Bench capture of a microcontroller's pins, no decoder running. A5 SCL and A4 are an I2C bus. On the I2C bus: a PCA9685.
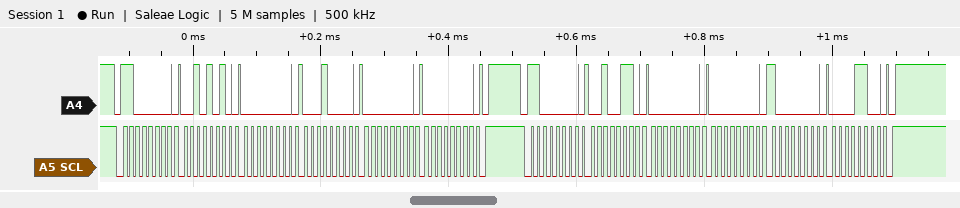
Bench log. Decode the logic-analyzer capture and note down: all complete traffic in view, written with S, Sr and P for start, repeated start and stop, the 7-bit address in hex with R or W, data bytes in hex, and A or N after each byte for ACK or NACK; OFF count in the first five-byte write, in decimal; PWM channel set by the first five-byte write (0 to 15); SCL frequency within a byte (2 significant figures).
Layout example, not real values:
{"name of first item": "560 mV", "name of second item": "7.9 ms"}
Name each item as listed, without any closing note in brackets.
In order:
{"all complete traffic in view, written with S, Sr and P for start, repeated start and stop, the 7-bit address in hex with R or W, data bytes in hex, and A or N after each byte for ACK or NACK": "S 60W A 2A A 00 A 10 A 00 A 00 A P S 60W A 26 A 00 A 00 A 80 A 0C A P", "OFF count in the first five-byte write, in decimal": "0", "PWM channel set by the first five-byte write": "9", "SCL frequency within a byte": "100 kHz"}
